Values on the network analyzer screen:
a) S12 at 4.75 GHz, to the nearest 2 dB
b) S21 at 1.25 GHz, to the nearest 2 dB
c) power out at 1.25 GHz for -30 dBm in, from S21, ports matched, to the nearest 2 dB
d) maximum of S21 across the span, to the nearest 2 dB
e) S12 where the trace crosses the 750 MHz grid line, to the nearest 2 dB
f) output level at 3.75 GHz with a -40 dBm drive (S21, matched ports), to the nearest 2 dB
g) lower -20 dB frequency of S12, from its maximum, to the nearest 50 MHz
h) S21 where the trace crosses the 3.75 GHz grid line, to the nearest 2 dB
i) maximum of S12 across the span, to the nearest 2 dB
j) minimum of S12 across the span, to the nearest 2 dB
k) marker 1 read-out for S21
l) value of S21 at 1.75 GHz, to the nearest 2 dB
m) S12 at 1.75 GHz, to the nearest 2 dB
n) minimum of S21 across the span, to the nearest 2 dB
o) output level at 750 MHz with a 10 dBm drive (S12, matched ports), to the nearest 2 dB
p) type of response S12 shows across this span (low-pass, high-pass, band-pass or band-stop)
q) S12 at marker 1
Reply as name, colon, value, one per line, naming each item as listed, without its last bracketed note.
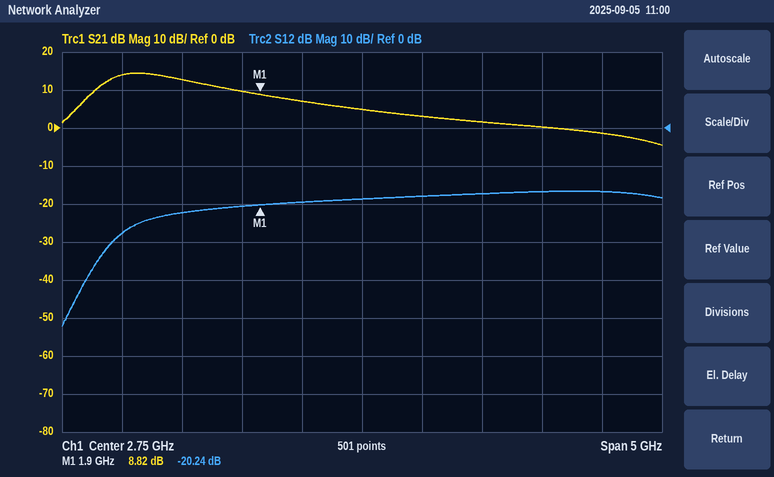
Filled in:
S12 at 4.75 GHz, to the nearest 2 dB: -16 dB
S21 at 1.25 GHz, to the nearest 2 dB: 12 dB
power out at 1.25 GHz for -30 dBm in, from S21, ports matched, to the nearest 2 dB: -18 dBm
maximum of S21 across the span, to the nearest 2 dB: 14 dB
S12 where the trace crosses the 750 MHz grid line, to the nearest 2 dB: -28 dB
output level at 3.75 GHz with a -40 dBm drive (S21, matched ports), to the nearest 2 dB: -38 dBm
lower -20 dB frequency of S12, from its maximum, to the nearest 50 MHz: 500 MHz
S21 where the trace crosses the 3.75 GHz grid line, to the nearest 2 dB: 2 dB
maximum of S12 across the span, to the nearest 2 dB: -16 dB
minimum of S12 across the span, to the nearest 2 dB: -52 dB
marker 1 read-out for S21: 8.82 dB
value of S21 at 1.75 GHz, to the nearest 2 dB: 10 dB
S12 at 1.75 GHz, to the nearest 2 dB: -20 dB
minimum of S21 across the span, to the nearest 2 dB: -4 dB
output level at 750 MHz with a 10 dBm drive (S12, matched ports), to the nearest 2 dB: -18 dBm
type of response S12 shows across this span: high-pass
S12 at marker 1: -20.24 dB
